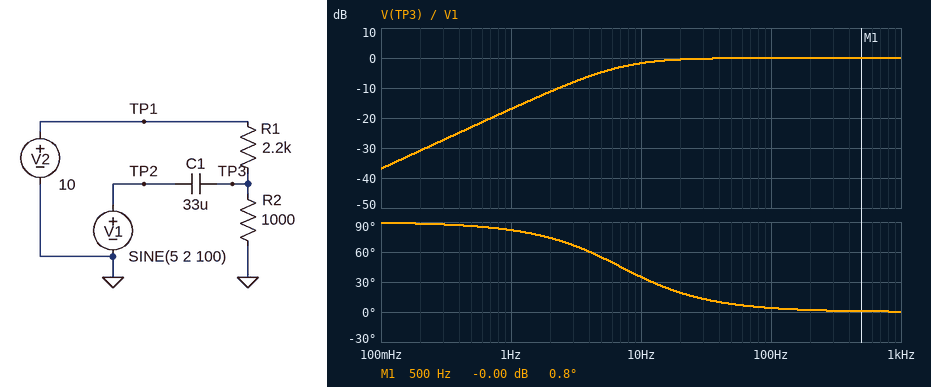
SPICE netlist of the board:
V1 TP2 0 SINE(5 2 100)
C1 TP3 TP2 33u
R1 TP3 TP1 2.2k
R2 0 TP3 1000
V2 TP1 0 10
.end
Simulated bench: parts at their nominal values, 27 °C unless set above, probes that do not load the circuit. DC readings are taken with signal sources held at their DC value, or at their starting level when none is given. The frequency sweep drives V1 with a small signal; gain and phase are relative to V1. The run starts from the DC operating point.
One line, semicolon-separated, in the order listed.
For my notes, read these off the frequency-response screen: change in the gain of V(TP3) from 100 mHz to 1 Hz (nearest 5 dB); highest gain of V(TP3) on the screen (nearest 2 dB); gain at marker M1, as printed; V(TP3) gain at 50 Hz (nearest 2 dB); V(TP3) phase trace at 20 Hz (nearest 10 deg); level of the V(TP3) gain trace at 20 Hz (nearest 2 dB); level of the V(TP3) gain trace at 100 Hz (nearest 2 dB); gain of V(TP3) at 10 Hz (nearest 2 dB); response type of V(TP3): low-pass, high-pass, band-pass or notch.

20 dB; 0 dB; -0.00 dB; 0 dB; 20 deg; 0 dB; 0 dB; -2 dB; high-pass
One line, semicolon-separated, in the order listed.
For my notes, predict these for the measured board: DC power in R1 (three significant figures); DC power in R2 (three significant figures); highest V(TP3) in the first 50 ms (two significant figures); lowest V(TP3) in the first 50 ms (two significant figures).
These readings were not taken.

21.5 mW; 9.77 mW; 5.1 V; 1.0 V
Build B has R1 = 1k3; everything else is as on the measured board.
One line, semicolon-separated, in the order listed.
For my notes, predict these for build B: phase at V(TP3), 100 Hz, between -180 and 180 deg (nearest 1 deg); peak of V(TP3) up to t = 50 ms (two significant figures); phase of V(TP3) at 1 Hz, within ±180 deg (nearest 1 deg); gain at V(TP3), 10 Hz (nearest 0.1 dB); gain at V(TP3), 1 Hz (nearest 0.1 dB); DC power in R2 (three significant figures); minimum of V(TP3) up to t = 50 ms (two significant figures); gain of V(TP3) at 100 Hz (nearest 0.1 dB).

5 deg; 6.3 V; 83 deg; -2.4 dB; -18.7 dB; 18.9 mW; 2.2 V; 0 dB
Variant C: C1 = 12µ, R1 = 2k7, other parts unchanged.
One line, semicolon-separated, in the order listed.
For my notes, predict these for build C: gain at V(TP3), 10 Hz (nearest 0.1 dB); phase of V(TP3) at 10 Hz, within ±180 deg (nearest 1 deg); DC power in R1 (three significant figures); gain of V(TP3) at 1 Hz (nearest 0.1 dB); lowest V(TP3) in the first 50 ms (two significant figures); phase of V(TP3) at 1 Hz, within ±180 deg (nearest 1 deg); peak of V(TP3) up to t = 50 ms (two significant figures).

-6.3 dB; 61 deg; 19.7 mW; -25.2 dB; 580 mV; 87 deg; 4.7 V
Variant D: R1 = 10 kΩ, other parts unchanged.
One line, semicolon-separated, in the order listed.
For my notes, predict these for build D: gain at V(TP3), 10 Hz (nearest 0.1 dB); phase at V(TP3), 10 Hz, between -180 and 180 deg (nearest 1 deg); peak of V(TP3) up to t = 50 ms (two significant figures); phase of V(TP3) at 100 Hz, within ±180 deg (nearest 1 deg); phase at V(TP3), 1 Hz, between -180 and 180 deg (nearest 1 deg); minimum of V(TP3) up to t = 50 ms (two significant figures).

-1.1 dB; 28 deg; 2.9 V; 3 deg; 79 deg; -1.2 V
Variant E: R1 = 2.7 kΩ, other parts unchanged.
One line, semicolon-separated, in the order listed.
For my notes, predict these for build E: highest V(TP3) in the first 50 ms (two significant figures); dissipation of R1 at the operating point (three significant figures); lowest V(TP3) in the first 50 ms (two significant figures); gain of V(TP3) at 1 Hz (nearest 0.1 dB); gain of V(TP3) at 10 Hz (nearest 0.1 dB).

4.7 V; 19.7 mW; 610 mV; -16.5 dB; -1.6 dB
